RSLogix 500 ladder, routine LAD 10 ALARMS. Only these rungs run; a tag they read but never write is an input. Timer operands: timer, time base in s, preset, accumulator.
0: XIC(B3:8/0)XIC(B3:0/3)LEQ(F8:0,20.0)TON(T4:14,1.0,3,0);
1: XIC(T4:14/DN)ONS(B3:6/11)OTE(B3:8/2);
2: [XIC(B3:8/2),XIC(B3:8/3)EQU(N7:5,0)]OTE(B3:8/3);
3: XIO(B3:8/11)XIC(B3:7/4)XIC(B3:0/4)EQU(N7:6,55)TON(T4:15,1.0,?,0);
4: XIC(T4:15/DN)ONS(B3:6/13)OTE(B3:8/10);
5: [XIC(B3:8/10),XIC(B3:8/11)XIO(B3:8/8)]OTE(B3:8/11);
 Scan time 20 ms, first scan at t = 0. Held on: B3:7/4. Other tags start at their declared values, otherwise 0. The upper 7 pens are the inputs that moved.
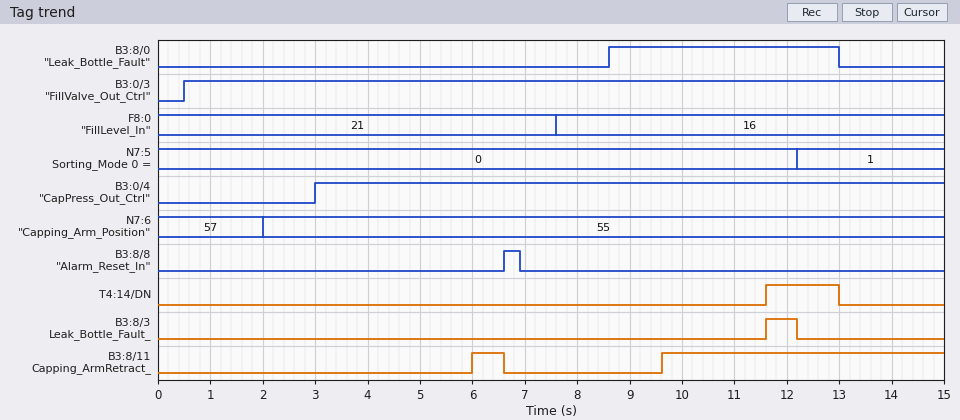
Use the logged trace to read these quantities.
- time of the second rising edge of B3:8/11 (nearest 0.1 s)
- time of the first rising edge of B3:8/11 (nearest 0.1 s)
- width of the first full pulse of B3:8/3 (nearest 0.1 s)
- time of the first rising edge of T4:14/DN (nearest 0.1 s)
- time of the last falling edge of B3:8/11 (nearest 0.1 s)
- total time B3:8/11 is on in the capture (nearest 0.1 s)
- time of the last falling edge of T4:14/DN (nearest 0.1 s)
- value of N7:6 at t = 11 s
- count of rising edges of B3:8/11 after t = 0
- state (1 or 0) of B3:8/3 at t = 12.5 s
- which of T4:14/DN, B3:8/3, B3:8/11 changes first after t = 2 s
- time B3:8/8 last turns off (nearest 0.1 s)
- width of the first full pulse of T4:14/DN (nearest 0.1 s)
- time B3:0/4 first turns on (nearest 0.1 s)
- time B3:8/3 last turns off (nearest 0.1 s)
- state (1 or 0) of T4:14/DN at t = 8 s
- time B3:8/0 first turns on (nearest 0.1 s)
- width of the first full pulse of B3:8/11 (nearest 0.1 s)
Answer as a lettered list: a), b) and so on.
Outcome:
a) 9.6 s
b) 6.0 s
c) 0.6 s
d) 11.6 s
e) 6.6 s
f) 6.0 s
g) 13.0 s
h) 55
i) 2
j) 0
k) B3:8/11
l) 6.9 s
m) 1.4 s
n) 3.0 s
o) 12.2 s
p) 0
q) 8.6 s
r) 0.6 s
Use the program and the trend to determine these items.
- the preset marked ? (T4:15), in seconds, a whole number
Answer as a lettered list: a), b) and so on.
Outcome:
a) 3 s
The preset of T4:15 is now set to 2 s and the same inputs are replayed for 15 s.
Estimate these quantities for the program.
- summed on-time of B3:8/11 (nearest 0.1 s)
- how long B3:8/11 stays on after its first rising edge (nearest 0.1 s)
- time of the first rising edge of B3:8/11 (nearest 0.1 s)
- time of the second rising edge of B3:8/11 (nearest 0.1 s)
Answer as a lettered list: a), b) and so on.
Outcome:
a) 8.0 s
b) 1.6 s
c) 5.0 s
d) 8.6 s
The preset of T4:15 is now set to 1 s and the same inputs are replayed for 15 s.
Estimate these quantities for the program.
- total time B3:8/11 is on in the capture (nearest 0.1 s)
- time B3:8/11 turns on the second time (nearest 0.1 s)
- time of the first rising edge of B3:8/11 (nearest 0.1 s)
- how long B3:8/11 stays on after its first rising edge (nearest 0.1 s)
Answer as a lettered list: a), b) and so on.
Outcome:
a) 10.0 s
b) 7.6 s
c) 4.0 s
d) 2.6 s
